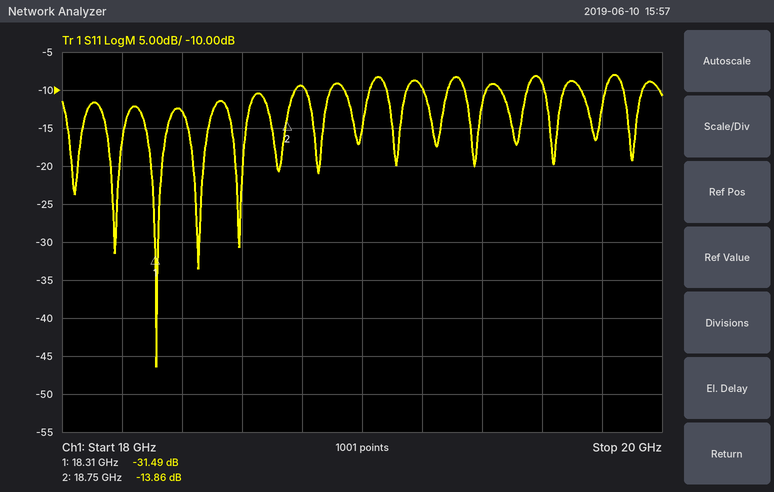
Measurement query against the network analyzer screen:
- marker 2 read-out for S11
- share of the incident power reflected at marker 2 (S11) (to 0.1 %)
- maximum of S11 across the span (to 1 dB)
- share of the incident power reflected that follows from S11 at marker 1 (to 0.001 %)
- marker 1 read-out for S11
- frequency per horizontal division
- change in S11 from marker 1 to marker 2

-13.86 dB
4.1 %
-8 dB
0.071 %
-31.49 dB
200 MHz
17.63 dB
